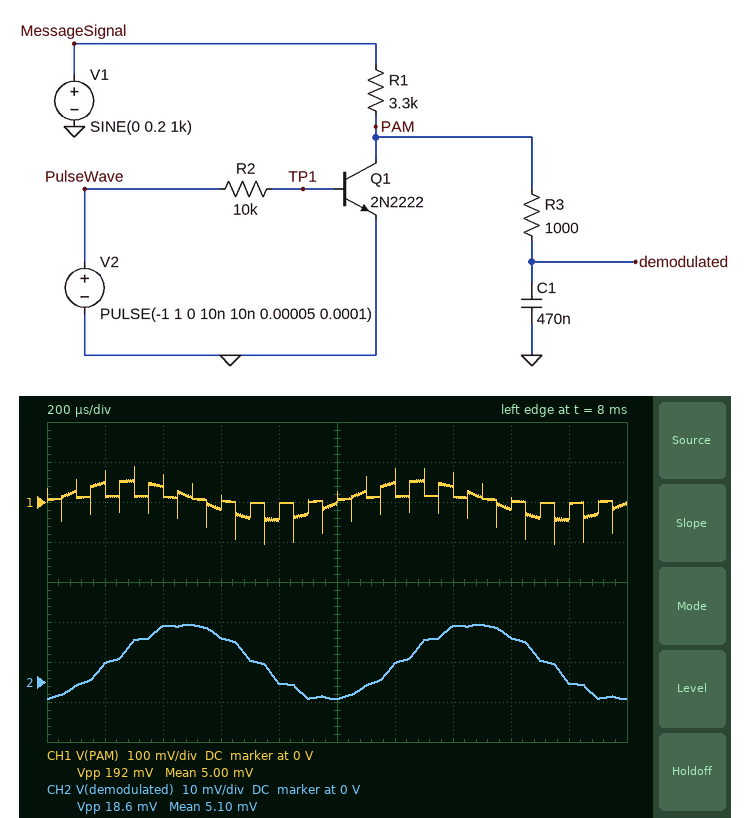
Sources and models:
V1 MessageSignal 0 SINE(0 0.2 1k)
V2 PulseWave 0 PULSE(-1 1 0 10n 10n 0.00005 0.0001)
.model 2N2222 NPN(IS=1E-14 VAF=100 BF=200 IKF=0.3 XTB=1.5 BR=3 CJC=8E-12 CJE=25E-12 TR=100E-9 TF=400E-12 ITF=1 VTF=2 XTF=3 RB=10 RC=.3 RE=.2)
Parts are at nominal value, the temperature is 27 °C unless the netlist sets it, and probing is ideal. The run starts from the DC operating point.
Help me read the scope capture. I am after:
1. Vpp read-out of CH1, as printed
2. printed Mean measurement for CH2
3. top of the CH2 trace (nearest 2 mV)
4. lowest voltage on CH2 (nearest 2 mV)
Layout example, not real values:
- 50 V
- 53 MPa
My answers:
- 192 mV
- 5.10 mV
- 14 mV
- -4 mV
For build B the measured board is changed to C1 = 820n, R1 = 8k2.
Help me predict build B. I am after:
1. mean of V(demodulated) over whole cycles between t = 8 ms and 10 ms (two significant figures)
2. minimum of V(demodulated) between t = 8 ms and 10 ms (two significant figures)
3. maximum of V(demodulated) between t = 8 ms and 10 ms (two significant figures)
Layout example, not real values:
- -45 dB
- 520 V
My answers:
- 6.3 mV
- 3.8 mV
- 8.8 mV
